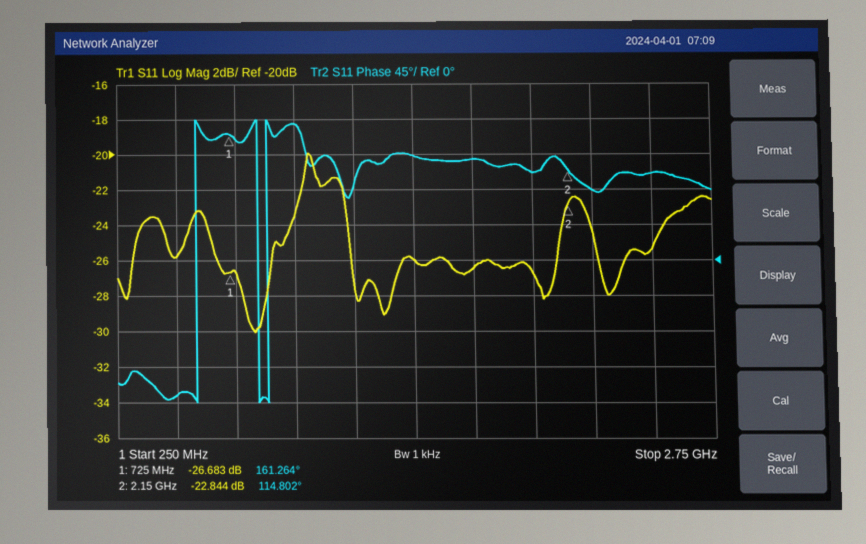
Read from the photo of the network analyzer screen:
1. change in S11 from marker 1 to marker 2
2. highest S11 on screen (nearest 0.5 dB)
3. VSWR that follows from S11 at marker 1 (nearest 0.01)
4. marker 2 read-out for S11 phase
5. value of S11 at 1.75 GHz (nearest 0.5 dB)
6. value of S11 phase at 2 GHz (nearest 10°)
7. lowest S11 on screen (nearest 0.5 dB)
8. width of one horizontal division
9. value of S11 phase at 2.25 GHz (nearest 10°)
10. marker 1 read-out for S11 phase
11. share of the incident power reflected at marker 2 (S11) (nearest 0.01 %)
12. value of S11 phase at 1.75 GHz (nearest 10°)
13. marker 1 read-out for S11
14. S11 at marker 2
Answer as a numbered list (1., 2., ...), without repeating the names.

1. 3.839 dB
2. -20.0 dB
3. 1.10
4. 114.802°
5. -26.5 dB
6. 110°
7. -30.0 dB
8. 250 MHz
9. 90°
10. 161.264°
11. 0.52 %
12. 130°
13. -26.683 dB
14. -22.844 dB
